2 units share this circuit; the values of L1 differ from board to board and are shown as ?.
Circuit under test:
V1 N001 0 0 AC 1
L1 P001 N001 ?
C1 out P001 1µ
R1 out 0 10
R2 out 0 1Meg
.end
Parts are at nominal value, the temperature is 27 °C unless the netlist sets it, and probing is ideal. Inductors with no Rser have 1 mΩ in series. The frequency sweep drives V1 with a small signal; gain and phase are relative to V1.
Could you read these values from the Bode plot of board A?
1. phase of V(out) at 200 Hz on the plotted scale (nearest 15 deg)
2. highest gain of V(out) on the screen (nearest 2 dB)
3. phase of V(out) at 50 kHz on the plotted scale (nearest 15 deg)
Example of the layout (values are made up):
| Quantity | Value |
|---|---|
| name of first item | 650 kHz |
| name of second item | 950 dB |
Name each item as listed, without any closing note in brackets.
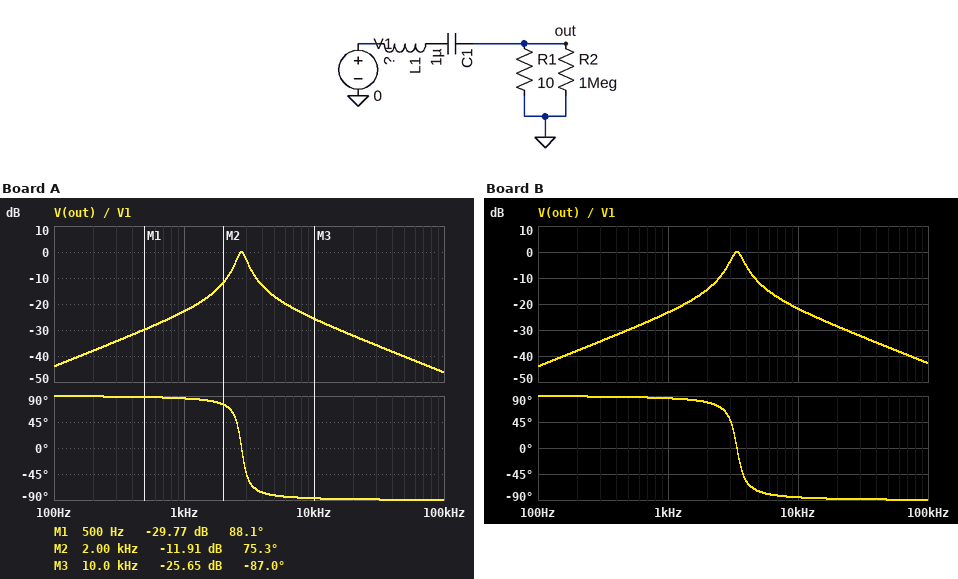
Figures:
| Quantity | Value |
|---|---|
| phase of V(out) at 200 Hz on the plotted scale | 90 deg |
| highest gain of V(out) on the screen | 0 dB |
| phase of V(out) at 50 kHz on the plotted scale | -90 deg |
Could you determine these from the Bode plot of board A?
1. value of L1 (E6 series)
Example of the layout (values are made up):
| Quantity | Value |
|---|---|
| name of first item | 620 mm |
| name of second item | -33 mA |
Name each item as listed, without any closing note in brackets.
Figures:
| Quantity | Value |
|---|---|
| value of L1 | 3.3 mH |
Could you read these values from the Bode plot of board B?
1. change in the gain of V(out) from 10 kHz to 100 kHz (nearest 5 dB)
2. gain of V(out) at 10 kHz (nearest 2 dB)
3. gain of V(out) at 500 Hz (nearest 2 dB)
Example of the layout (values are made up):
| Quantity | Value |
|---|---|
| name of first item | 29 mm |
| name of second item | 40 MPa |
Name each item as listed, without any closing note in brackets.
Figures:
| Quantity | Value |
|---|---|
| change in the gain of V(out) from 10 kHz to 100 kHz | -20 dB |
| gain of V(out) at 10 kHz | -22 dB |
| gain of V(out) at 500 Hz | -30 dB |
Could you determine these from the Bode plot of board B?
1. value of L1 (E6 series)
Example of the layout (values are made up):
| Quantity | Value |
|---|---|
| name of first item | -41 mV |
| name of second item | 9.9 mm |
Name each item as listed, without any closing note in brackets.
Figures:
| Quantity | Value |
|---|---|
| value of L1 | 2.2 mH |
